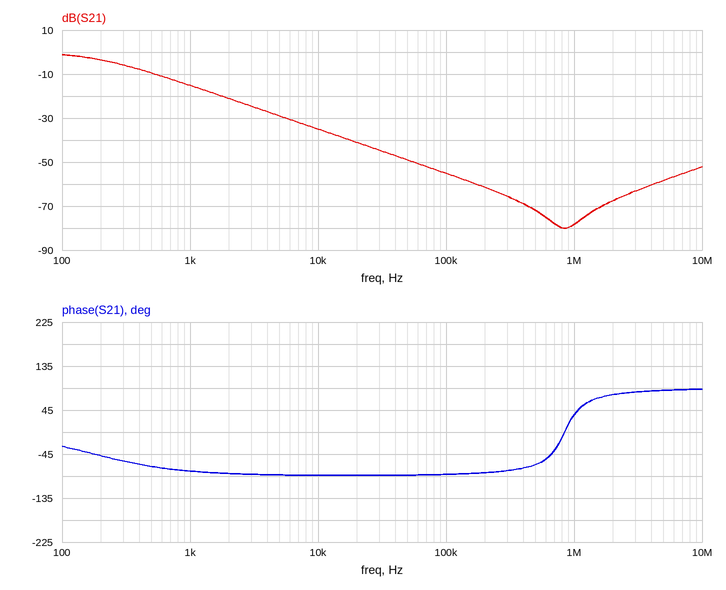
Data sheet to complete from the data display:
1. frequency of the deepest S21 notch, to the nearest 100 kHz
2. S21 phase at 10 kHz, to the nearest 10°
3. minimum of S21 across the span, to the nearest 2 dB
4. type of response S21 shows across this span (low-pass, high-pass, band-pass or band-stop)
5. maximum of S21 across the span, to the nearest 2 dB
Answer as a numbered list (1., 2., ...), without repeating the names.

1. 800 kHz
2. -90°
3. -80 dB
4. low-pass
5. -2 dB
